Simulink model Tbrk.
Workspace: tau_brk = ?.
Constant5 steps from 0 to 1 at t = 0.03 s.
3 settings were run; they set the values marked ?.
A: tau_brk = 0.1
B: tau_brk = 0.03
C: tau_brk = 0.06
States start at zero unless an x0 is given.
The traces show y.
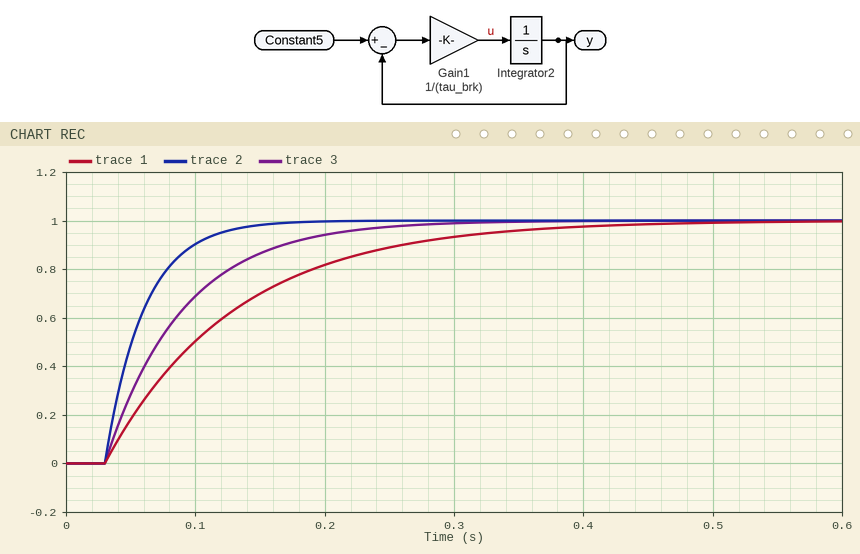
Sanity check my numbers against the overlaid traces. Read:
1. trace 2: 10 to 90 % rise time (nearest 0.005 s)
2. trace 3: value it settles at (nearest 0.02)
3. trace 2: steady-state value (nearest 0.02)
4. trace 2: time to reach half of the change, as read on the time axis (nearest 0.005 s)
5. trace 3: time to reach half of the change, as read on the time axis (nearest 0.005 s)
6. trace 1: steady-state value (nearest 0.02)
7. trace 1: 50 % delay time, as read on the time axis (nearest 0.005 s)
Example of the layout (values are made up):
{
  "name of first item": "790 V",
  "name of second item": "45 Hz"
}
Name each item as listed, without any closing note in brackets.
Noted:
{
  "trace 2: 10 to 90 % rise time": "0.065 s",
  "trace 3: value it settles at": "1.00",
  "trace 2: steady-state value": "1.00",
  "trace 2: time to reach half of the change, as read on the time axis": "0.050 s",
  "trace 3: time to reach half of the change, as read on the time axis": "0.070 s",
  "trace 1: steady-state value": "1.00",
  "trace 1: 50 % delay time, as read on the time axis": "0.100 s"
}
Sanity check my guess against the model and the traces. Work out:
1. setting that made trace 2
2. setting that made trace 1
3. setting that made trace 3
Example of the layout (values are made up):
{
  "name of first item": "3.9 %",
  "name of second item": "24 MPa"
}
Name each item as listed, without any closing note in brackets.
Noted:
{
  "setting that made trace 2": "B",
  "setting that made trace 1": "A",
  "setting that made trace 3": "C"
}
